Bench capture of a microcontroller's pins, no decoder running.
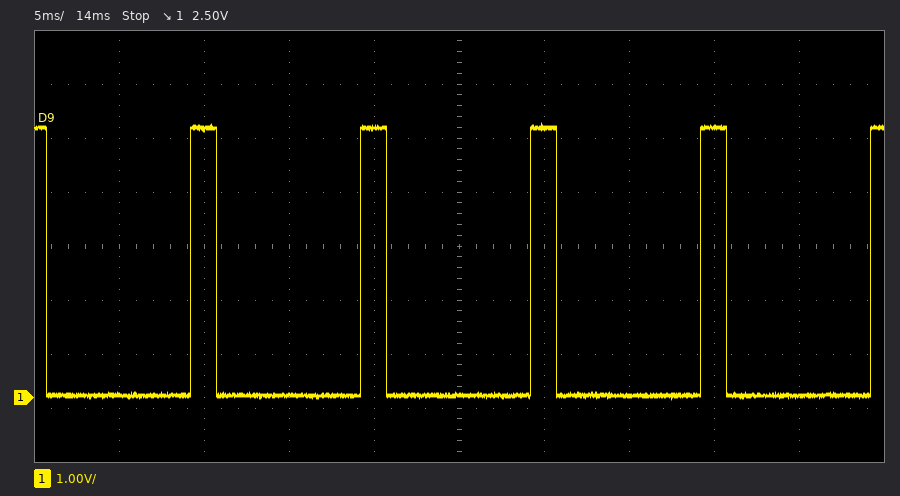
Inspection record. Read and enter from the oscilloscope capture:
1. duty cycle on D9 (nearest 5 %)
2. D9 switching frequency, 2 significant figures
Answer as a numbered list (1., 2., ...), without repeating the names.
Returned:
1. 15 %
2. 100 Hz
